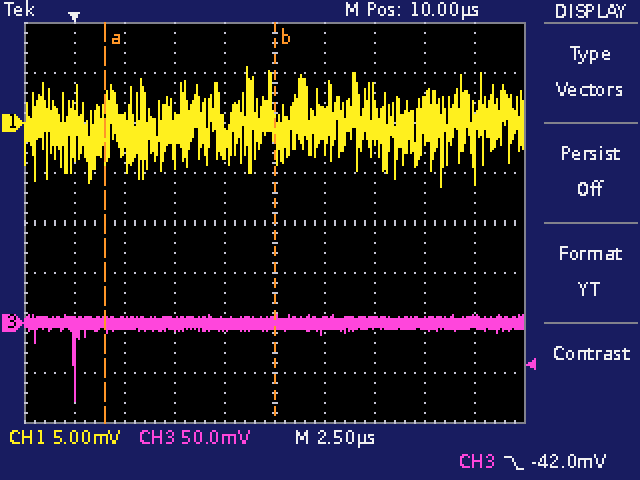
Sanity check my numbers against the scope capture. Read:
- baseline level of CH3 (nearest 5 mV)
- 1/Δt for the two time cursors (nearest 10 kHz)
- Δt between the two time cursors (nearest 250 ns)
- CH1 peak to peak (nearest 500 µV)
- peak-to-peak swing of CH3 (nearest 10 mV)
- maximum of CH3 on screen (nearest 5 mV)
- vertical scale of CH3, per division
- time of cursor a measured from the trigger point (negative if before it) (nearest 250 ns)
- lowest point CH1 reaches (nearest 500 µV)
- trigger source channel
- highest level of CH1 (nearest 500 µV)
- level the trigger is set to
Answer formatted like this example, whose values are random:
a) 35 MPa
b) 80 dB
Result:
a) 0 mV
b) 120 kHz
c) 8.50 µs
d) 12.0 mV
e) 90 mV
f) 10 mV
g) 50 mV
h) +1.50 µs
i) -6.5 mV
j) CH3
k) 5.5 mV
l) -42.0 mV
